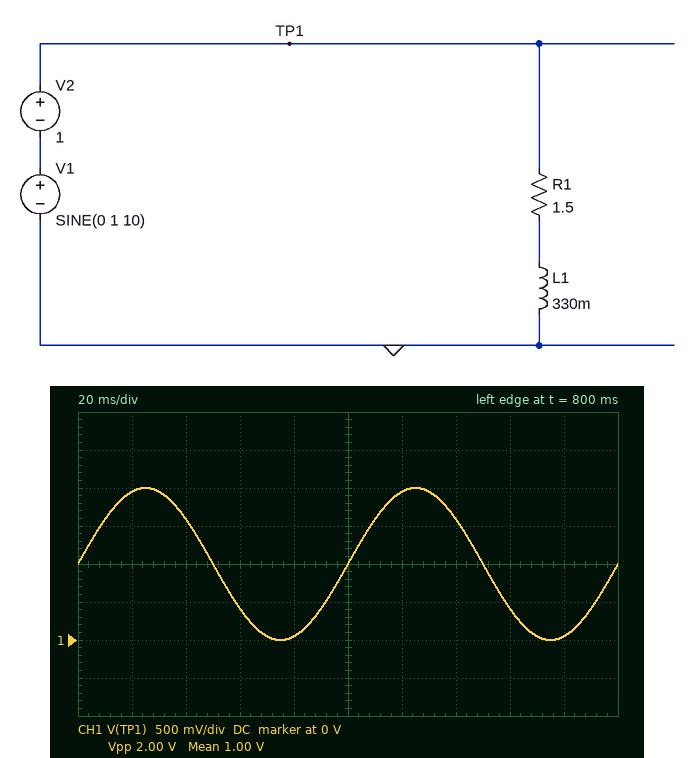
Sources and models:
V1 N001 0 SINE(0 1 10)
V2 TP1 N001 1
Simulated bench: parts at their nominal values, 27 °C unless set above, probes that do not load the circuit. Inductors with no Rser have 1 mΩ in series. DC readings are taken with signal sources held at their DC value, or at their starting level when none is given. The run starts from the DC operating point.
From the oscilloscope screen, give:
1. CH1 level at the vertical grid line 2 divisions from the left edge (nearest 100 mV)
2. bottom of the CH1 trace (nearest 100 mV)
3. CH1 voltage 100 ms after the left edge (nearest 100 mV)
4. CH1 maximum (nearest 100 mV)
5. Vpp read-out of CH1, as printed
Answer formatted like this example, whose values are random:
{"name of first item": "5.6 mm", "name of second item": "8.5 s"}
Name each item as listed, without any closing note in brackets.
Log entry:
{"CH1 level at the vertical grid line 2 divisions from the left edge": "1.6 V", "bottom of the CH1 trace": "0 V", "CH1 voltage 100 ms after the left edge": "1.0 V", "CH1 maximum": "2.0 V", "Vpp read-out of CH1, as printed": "2.00 V"}
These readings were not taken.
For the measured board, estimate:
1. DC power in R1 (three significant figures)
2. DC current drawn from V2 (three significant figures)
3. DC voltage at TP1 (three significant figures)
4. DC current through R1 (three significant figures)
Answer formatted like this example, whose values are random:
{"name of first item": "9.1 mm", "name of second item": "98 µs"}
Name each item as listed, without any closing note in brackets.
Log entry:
{"DC power in R1": "666 mW", "DC current drawn from V2": "666 mA", "DC voltage at TP1": "1.00 V", "DC current through R1": "666 mA"}
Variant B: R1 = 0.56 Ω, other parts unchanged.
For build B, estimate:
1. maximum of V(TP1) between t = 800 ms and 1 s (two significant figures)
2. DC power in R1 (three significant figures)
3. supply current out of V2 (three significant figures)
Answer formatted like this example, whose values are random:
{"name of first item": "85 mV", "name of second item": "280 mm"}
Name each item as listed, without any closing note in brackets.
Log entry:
{"maximum of V(TP1) between t = 800 ms and 1 s": "2.0 V", "DC power in R1": "1.78 W", "supply current out of V2": "1.78 A"}
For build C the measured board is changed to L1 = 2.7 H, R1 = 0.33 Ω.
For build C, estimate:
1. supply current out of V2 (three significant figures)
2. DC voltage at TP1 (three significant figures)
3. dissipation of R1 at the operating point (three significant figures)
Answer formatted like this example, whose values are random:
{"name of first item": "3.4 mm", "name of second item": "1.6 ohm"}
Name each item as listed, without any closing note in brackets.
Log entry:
{"supply current out of V2": "3.02 A", "DC voltage at TP1": "1.00 V", "dissipation of R1 at the operating point": "3.01 W"}
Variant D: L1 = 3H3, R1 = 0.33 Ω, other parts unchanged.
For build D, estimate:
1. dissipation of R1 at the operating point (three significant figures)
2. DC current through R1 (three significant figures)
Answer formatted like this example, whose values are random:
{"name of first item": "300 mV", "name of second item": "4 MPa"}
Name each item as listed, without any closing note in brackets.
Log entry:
{"dissipation of R1 at the operating point": "3.01 W", "DC current through R1": "3.02 A"}
